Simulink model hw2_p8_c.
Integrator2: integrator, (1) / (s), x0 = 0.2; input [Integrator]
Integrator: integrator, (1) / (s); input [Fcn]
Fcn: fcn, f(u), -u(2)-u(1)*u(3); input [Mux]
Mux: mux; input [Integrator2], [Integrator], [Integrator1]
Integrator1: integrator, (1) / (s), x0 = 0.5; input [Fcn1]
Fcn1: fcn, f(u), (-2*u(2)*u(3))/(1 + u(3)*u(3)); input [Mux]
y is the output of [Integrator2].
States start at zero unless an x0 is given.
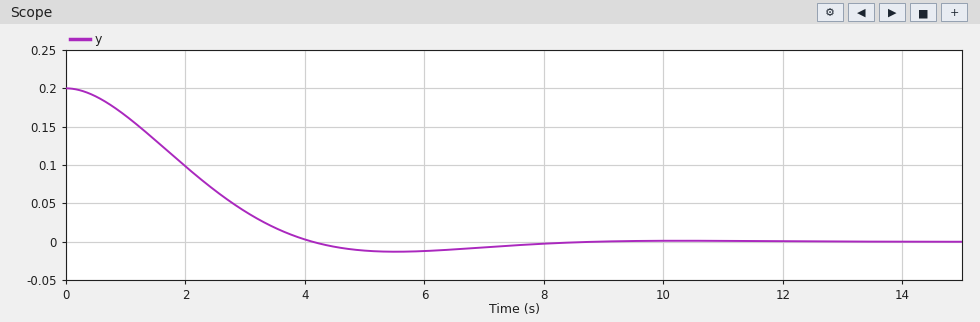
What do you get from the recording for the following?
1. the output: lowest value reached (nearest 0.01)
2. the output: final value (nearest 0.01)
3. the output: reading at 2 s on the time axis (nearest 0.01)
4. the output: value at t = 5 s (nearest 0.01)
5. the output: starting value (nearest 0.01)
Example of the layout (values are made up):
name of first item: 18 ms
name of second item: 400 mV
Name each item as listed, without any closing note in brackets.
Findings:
the output: lowest value reached: -0.01
the output: final value: 0.00
the output: reading at 2 s on the time axis: 0.10
the output: value at t = 5 s: -0.01
the output: starting value: 0.20
